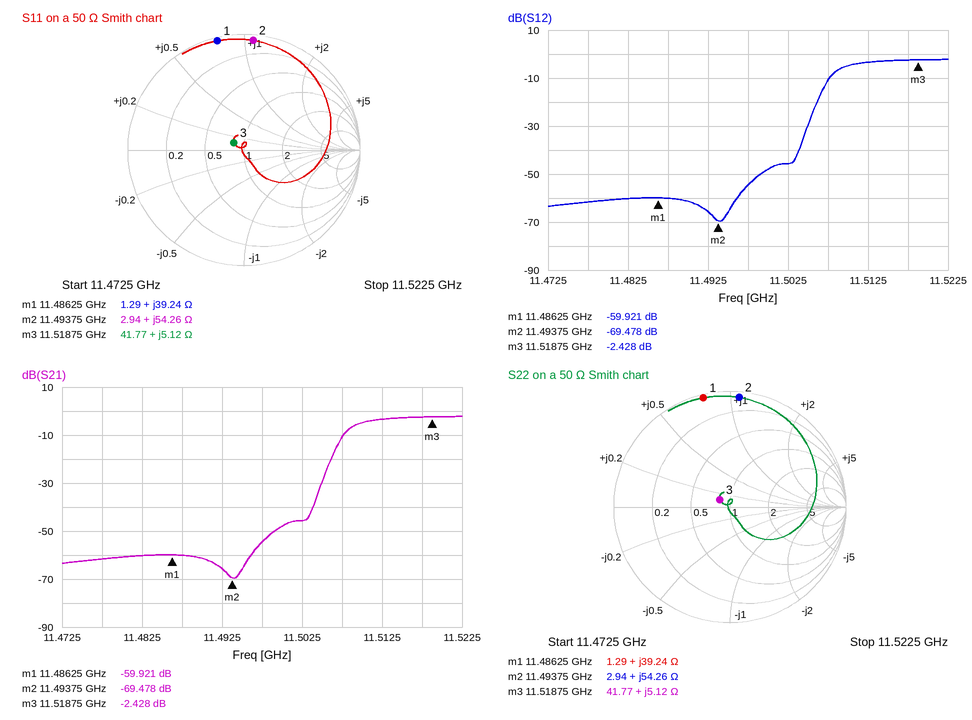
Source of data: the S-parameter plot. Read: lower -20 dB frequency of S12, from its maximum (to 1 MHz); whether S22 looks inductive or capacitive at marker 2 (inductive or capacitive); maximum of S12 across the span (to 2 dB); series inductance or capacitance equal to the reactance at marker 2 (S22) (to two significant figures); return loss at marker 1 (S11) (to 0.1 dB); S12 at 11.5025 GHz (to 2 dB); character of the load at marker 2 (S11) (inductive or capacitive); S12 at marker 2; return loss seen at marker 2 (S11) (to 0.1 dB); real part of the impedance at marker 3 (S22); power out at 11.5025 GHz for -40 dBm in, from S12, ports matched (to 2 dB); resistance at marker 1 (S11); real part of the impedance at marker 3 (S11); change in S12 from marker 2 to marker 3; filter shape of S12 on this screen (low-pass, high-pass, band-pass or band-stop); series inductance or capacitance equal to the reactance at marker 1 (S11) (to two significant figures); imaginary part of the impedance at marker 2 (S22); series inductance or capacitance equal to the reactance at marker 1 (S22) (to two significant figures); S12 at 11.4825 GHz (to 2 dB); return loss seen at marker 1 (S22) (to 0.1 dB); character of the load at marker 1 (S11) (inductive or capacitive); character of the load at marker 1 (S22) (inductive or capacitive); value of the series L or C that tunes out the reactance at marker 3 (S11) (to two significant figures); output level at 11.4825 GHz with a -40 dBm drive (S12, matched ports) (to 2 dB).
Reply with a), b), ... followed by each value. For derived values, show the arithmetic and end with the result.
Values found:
a) 11.506 GHz
b) inductive
c) -2 dB
d) L = 54.26 Ω/(2π × 11.49375 GHz) ≈ 751 pH, so 750 pH to two significant figures
e) 0.3 dB
f) -46 dB
g) inductive
h) -69.478 dB
i) 0.5 dB
j) 41.77 Ω
k) -40 dBm + (-46 dB) = -86 dBm
l) 1.29 Ω
m) 41.77 Ω
n) -2.428 − (-69.478) = 67.050 dB
o) high-pass
p) L = 39.24 Ω/(2π × 11.48625 GHz) ≈ 544 pH, so 540 pH to two significant figures
q) +54.26 Ω
r) L = 39.24 Ω/(2π × 11.48625 GHz) ≈ 544 pH, so 540 pH to two significant figures
s) -60 dB
t) 0.3 dB
u) inductive
v) inductive
w) C = 1/(2π × 11.51875 GHz × 5.12 Ω) ≈ 2.7 pF
x) -40 dBm + (-60 dB) = -100 dBm
